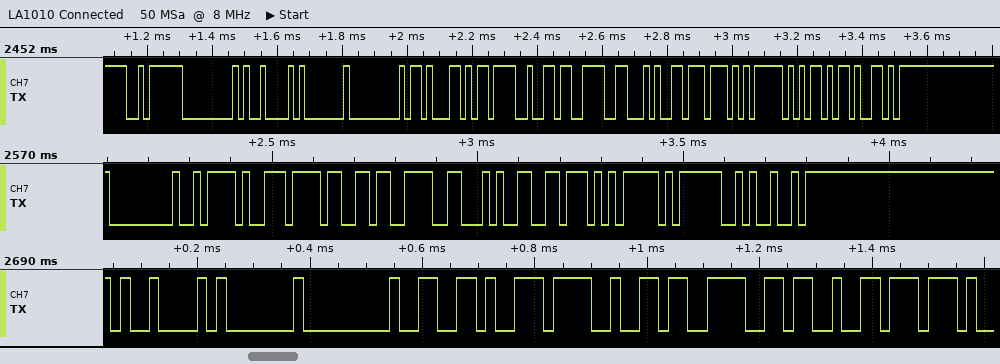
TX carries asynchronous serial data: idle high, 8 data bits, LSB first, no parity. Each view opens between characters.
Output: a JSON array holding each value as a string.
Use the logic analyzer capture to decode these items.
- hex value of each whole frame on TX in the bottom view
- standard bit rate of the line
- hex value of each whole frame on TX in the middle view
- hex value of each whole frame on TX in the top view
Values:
["09, 01, 00, 66, EE, B2, 9E, 93, 77", "57600 baud", "00, 7A, EE, B3, 9E, 94, 76, 7D, 3F, 49", "FA, 00, 09, 01, 00, 8B, ED, B2, 9E, 94, 77, 7D, AD, 59"]
